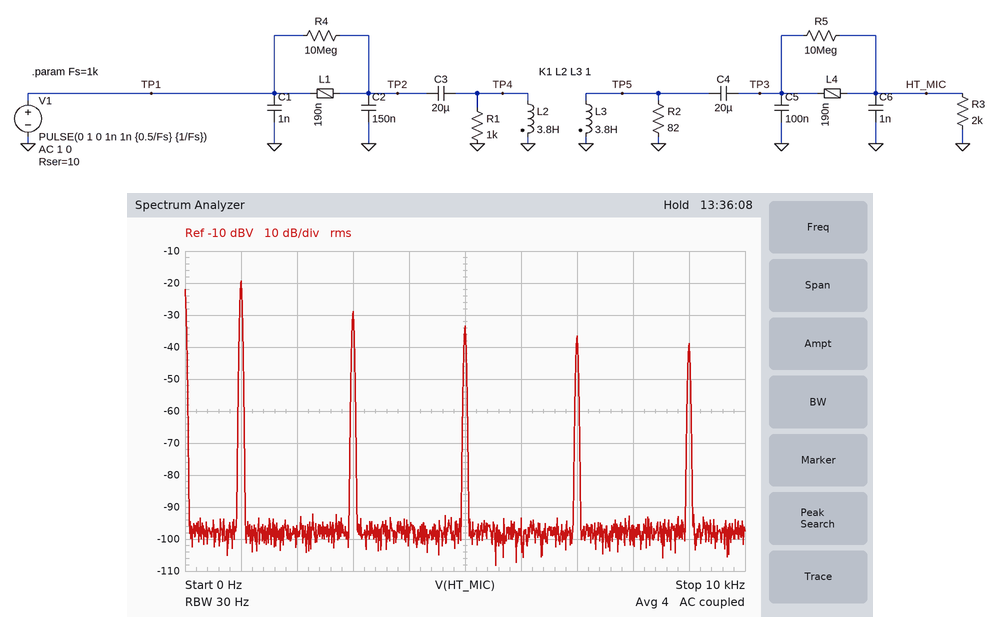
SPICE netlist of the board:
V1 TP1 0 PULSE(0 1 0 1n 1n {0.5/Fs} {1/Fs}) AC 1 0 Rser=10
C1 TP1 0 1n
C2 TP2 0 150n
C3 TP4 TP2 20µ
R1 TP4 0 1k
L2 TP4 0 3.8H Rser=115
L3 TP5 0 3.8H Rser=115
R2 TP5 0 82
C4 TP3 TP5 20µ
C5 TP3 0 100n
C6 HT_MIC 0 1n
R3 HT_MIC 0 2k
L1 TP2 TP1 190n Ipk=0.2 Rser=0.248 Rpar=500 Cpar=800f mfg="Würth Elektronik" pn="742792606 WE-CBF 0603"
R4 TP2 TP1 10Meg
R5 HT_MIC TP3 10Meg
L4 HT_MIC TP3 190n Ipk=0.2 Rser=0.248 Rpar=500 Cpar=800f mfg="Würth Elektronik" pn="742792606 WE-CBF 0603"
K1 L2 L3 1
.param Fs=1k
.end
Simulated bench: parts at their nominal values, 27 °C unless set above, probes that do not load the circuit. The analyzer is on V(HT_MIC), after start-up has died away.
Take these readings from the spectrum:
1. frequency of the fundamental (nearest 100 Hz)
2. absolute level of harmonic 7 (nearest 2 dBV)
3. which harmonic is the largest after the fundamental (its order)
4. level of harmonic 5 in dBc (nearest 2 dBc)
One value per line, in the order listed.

1.0 kHz
-36 dBV
3
-14 dBc
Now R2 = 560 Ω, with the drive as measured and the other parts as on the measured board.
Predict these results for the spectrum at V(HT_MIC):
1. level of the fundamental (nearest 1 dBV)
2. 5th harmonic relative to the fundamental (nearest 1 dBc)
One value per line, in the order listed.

-11 dBV
-15 dBc
